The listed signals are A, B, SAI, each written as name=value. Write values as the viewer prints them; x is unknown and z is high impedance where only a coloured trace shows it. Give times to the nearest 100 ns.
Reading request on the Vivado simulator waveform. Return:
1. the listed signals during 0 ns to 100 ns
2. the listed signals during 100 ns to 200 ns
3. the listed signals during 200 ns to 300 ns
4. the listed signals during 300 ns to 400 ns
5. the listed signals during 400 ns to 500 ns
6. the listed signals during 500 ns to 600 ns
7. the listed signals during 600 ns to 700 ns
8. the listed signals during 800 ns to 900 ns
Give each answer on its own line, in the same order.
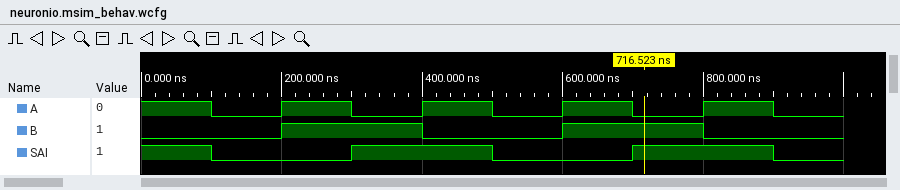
A=1, B=0, SAI=1
A=0, B=0, SAI=0
A=1, B=1, SAI=0
A=0, B=1, SAI=1
A=1, B=0, SAI=1
A=0, B=0, SAI=0
A=1, B=1, SAI=0
A=1, B=0, SAI=1
